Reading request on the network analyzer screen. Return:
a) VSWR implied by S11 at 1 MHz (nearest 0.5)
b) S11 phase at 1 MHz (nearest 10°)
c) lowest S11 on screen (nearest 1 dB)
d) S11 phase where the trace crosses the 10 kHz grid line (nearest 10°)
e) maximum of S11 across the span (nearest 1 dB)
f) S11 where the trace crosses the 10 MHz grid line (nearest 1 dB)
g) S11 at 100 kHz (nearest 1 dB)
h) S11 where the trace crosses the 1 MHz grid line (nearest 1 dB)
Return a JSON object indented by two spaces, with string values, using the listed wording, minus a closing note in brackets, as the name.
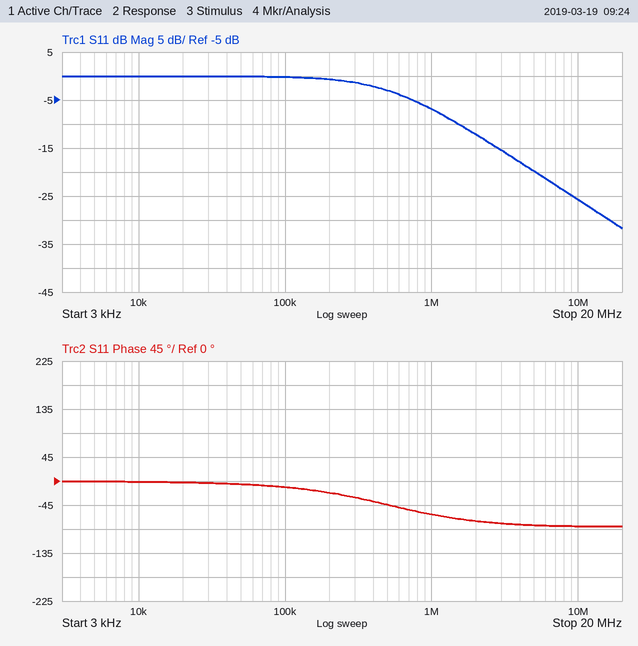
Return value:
{
  "VSWR implied by S11 at 1 MHz": "2.5",
  "S11 phase at 1 MHz": "-60°",
  "lowest S11 on screen": "-32 dB",
  "S11 phase where the trace crosses the 10 kHz grid line": "0°",
  "maximum of S11 across the span": "0 dB",
  "S11 where the trace crosses the 10 MHz grid line": "-26 dB",
  "S11 at 100 kHz": "0 dB",
  "S11 where the trace crosses the 1 MHz grid line": "-7 dB"
}
